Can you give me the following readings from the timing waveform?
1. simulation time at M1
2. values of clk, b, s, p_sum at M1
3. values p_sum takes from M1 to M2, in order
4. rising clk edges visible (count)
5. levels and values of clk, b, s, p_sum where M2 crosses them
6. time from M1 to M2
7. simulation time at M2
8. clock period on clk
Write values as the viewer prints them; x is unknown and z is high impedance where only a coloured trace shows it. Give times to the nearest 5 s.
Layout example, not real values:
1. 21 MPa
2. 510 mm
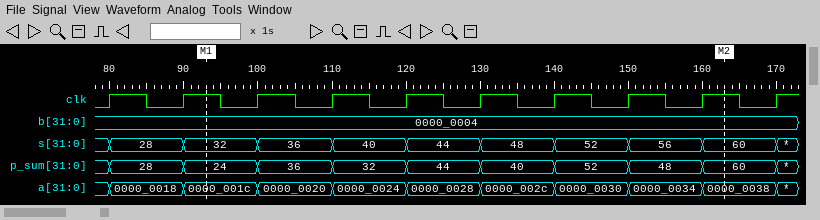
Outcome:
1. 95 s
2. clk=1, b=0000_0004, s=32, p_sum=24
3. 24, 36, 32, 44, 40, 52, 48, 60
4. 10
5. clk=1, b=0000_0004, s=60, p_sum=60
6. 70 s
7. 165 s
8. 10 s
